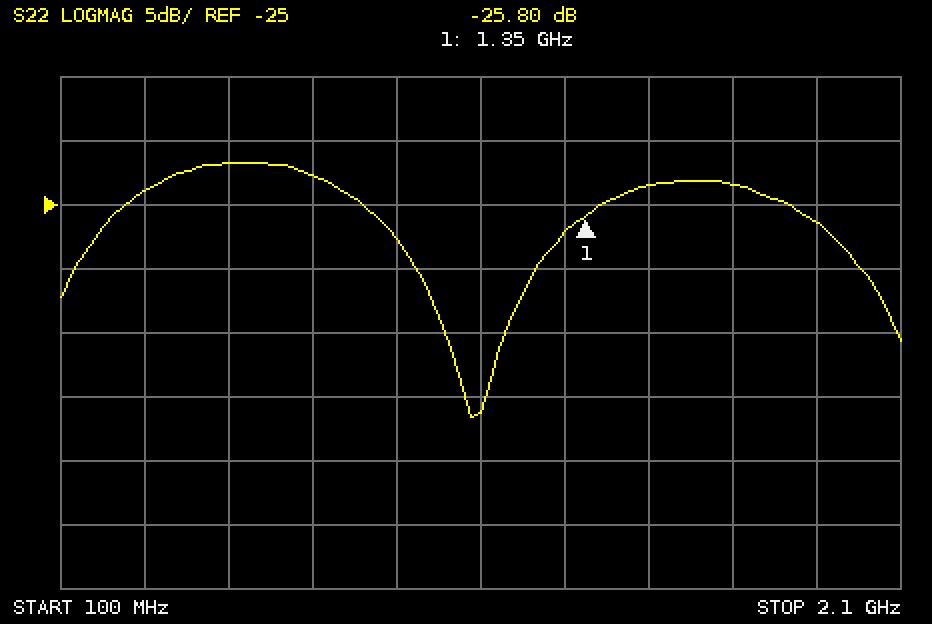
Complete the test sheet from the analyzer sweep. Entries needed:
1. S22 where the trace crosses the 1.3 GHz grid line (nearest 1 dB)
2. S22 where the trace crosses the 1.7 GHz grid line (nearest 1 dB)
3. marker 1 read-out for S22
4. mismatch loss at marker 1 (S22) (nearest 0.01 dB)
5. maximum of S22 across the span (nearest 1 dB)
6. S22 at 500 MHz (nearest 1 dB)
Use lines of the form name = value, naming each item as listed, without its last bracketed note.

S22 where the trace crosses the 1.3 GHz grid line = -27 dB
S22 where the trace crosses the 1.7 GHz grid line = -23 dB
marker 1 read-out for S22 = -25.80 dB
mismatch loss at marker 1 (S22) = 0.01 dB
maximum of S22 across the span = -22 dB
S22 at 500 MHz = -22 dB
